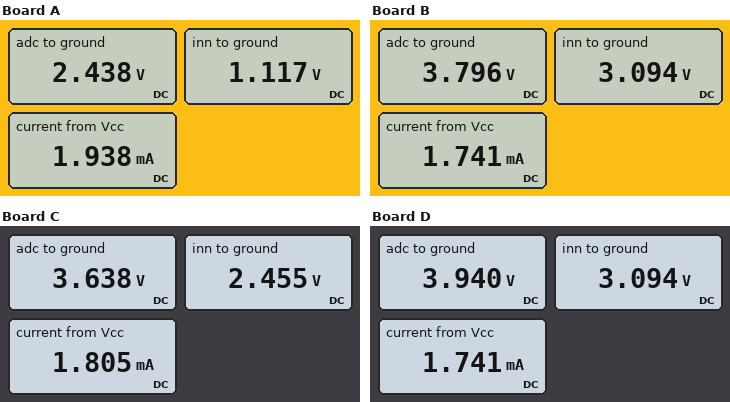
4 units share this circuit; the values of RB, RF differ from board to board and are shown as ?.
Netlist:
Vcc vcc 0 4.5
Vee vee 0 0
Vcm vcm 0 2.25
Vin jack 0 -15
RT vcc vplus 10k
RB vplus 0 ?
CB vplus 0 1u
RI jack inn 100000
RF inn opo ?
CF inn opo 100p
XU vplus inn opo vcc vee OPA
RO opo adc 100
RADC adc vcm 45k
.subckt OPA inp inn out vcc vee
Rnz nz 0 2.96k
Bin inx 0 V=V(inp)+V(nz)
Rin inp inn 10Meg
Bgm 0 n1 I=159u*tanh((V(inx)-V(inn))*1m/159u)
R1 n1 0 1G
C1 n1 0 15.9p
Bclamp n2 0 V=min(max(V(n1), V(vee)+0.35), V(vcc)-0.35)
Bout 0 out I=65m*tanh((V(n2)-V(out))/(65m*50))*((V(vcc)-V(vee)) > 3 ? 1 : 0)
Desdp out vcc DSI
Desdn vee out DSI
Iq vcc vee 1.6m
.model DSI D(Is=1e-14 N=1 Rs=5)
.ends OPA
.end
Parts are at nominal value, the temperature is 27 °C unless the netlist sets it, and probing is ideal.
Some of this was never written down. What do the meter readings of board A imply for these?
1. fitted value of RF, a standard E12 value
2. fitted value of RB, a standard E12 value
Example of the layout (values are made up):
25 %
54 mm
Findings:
8.2 kΩ
3.3 kΩ
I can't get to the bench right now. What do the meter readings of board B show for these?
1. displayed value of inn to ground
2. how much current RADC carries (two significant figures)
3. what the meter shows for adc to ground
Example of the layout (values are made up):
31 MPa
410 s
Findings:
3.094 V
34 µA
3.796 V
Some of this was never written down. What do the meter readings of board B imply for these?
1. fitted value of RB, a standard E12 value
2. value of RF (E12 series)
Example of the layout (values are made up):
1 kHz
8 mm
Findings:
22 kΩ
3.9 kΩ
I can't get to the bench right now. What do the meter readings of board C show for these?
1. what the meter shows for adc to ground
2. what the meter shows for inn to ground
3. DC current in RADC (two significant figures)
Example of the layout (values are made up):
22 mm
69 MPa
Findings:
3.638 V
2.455 V
31 µA
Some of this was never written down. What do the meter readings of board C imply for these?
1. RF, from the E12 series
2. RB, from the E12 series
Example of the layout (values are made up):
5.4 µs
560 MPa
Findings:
6.8 kΩ
12 kΩ
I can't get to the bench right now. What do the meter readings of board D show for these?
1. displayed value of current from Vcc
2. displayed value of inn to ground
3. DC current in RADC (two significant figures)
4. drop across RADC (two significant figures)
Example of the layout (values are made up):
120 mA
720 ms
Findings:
1.741 mA
3.094 V
38 µA
1.7 V
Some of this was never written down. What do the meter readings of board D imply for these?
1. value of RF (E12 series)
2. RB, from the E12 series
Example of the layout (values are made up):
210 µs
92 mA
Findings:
4.7 kΩ
22 kΩ
